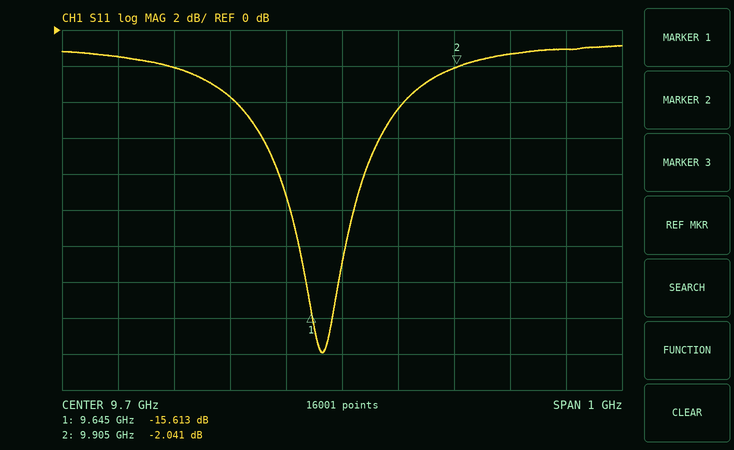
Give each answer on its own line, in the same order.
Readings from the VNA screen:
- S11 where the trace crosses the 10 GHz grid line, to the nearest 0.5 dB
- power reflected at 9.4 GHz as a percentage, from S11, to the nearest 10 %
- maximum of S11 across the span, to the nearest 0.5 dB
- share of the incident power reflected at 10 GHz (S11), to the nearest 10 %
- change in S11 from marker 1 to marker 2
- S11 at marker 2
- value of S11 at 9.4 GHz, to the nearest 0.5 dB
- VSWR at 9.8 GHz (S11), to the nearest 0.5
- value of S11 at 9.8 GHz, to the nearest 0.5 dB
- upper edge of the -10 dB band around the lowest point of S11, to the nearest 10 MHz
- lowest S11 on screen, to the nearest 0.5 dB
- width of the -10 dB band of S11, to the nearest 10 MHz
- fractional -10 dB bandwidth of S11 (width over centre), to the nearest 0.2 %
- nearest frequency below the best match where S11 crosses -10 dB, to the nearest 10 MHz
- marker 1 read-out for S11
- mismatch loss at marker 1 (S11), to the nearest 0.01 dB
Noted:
-1.5 dB
60 %
-1.0 dB
70 %
13.572 dB
-2.041 dB
-2.0 dB
4.0
-4.5 dB
9.72 GHz
-18.0 dB
110 MHz
1.2 %
9.61 GHz
-15.613 dB
0.12 dB
